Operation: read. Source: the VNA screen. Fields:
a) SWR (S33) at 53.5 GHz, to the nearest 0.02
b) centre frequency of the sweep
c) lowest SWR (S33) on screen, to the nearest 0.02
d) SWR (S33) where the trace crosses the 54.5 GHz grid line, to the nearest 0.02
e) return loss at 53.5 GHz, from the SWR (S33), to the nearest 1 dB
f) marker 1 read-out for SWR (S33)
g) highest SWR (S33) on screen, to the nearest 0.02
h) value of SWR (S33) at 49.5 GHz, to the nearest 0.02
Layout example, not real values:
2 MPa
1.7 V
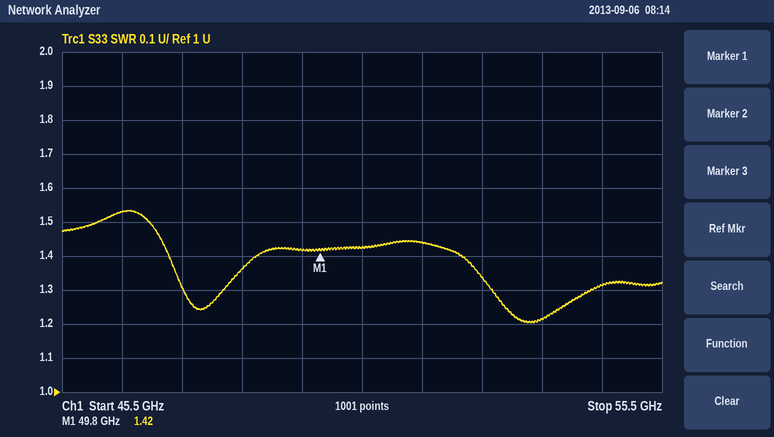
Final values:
1.22
50.5 GHz
1.20
1.32
20 dB
1.42
1.54
1.42
